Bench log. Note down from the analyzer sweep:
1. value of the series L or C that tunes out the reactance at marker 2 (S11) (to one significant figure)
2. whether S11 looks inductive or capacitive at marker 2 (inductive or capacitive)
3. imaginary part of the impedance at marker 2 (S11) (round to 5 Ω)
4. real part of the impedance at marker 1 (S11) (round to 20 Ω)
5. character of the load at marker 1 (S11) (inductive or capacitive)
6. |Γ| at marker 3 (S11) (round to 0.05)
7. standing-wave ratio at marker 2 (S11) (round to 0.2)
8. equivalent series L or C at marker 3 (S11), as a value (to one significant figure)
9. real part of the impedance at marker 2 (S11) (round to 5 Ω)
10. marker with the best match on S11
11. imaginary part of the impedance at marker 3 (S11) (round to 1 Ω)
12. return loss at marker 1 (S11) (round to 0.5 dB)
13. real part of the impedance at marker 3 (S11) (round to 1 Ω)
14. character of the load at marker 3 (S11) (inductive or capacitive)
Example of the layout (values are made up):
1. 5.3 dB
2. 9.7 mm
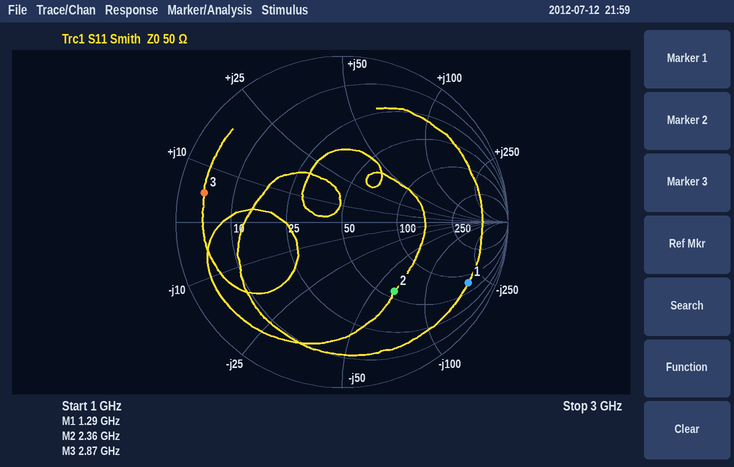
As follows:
1. 4 nH
2. capacitive
3. -65 Ω
4. 80 Ω
5. capacitive
6. 0.85
7. 3.2
8. 300 pH
9. 55 Ω
10. marker 2
11. +5 Ω
12. 1.5 dB
13. 4 Ω
14. inductive
